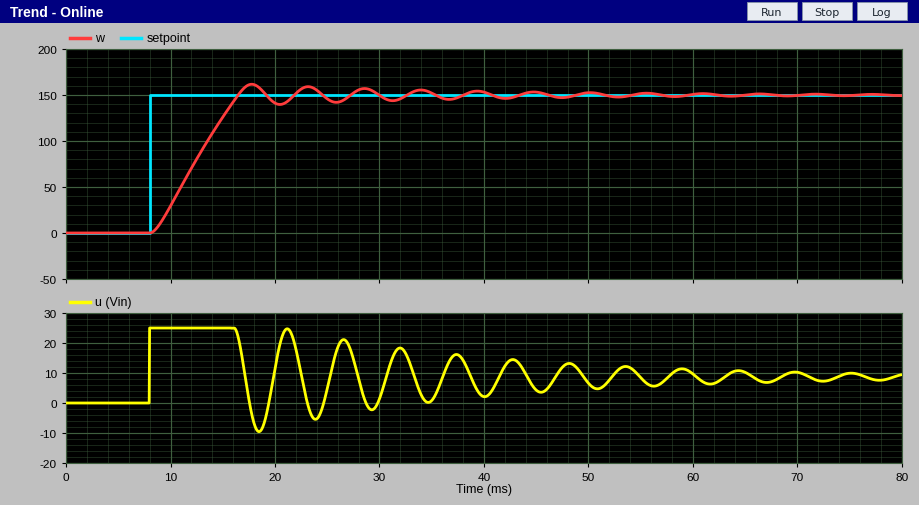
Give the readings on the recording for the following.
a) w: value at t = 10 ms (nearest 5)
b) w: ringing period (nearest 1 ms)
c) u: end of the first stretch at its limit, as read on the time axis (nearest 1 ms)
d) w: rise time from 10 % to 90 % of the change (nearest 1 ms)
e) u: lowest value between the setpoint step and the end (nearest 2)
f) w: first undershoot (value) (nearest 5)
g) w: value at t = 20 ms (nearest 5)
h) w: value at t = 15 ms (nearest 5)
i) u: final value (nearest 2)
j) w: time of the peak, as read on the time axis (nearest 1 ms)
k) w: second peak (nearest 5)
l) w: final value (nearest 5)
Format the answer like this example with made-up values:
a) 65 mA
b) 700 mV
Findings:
a) 30
b) 5 ms
c) 16 ms
d) 6 ms
e) -10
f) 140
g) 140
h) 125
i) 8
j) 18 ms
k) 160
l) 150
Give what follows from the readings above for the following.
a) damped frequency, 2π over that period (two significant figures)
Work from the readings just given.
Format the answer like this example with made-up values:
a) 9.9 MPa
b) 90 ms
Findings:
a) 1.3 rad/ms
